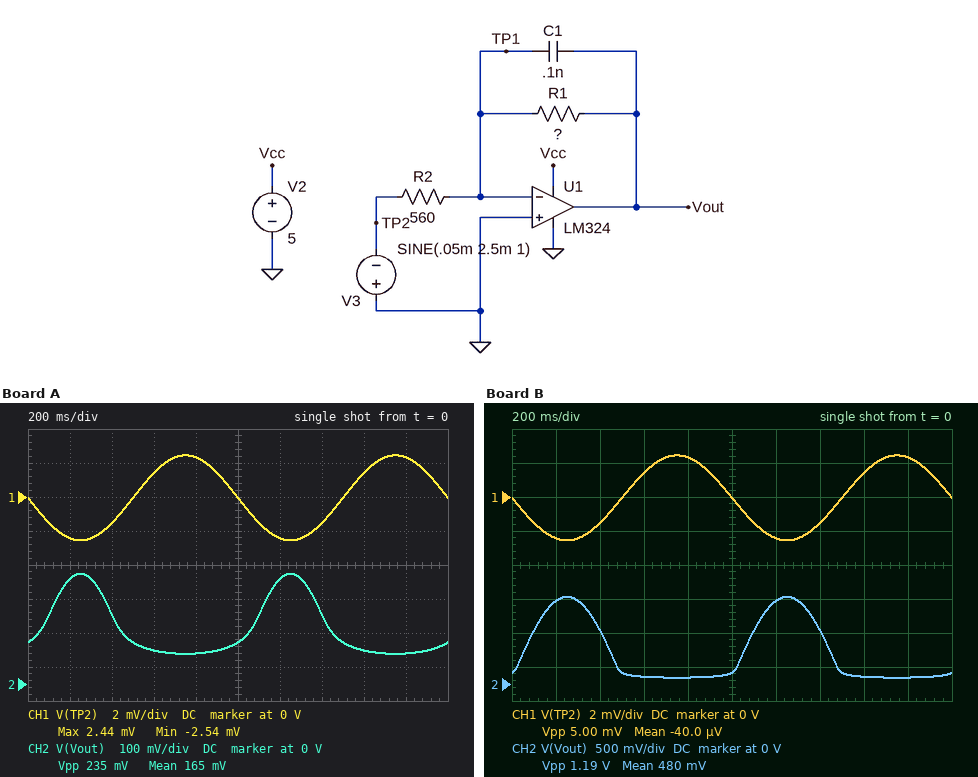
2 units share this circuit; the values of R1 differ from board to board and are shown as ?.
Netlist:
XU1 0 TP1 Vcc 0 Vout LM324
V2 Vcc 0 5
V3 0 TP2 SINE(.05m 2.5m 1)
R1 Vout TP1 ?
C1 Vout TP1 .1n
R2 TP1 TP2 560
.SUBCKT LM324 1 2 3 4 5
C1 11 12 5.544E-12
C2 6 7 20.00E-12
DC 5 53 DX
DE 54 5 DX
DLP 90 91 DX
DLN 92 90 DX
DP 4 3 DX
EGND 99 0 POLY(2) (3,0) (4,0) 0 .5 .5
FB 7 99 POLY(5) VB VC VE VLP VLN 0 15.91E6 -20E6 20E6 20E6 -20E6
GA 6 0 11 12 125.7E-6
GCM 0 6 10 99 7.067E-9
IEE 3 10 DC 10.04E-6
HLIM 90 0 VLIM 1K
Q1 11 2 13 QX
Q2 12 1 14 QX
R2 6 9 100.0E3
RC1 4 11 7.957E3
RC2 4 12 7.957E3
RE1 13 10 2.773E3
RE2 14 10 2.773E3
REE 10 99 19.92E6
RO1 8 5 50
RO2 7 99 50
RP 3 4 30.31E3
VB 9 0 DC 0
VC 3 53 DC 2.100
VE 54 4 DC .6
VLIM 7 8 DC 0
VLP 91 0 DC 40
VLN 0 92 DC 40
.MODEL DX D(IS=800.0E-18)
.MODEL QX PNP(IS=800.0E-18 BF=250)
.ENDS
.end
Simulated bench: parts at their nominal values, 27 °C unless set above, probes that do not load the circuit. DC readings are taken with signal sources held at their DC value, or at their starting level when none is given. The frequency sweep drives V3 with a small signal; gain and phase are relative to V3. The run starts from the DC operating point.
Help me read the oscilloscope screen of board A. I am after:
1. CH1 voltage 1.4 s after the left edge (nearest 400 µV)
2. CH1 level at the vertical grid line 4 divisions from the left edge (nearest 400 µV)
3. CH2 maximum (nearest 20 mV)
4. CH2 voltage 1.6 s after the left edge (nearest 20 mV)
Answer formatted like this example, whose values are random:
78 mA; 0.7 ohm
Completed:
-1.6 mV; 2.4 mV; 320 mV; 100 mV
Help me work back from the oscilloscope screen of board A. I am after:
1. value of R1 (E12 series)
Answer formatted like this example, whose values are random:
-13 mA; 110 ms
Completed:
68 kΩ
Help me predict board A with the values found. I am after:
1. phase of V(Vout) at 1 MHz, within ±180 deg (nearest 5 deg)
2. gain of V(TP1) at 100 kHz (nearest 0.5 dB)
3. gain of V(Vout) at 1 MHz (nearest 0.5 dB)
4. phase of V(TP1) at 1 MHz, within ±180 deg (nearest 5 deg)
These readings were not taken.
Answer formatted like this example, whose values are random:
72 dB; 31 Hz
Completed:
-130 deg; -2.0 dB; -5.5 dB; 170 deg
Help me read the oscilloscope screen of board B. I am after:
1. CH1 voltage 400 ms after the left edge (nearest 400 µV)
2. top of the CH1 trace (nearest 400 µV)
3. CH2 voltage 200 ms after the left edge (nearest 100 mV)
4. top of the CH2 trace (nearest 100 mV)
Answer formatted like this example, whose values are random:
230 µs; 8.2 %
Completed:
-1.6 mV; 2.4 mV; 1.2 V; 1.3 V
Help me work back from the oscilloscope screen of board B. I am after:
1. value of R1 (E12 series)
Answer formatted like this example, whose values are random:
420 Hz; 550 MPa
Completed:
270 kΩ
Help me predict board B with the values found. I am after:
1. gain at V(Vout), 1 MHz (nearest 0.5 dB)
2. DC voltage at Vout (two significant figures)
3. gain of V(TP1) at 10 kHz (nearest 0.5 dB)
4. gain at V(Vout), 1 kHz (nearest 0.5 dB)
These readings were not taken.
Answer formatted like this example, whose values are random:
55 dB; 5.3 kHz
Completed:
-3.5 dB; 160 mV; -2.5 dB; 41.0 dB
